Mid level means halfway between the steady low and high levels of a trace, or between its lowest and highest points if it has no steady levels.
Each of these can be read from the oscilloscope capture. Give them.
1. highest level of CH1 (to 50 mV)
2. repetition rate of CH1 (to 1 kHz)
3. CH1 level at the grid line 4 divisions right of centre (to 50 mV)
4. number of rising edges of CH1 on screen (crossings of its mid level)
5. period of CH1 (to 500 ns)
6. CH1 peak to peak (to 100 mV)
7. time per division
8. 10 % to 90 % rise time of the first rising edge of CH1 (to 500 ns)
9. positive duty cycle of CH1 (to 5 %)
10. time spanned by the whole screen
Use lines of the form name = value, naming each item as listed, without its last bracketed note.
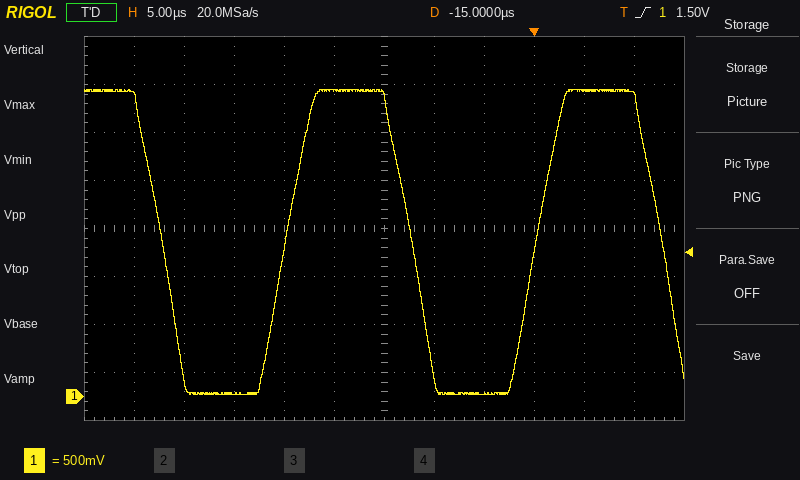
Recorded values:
highest level of CH1 = 3.20 V
repetition rate of CH1 = 40 kHz
CH1 level at the grid line 4 divisions right of centre = 3.20 V
number of rising edges of CH1 on screen = 2
period of CH1 = 25.0 µs
CH1 peak to peak = 3.20 V
time per division = 5 µs
10 % to 90 % rise time of the first rising edge of CH1 = 4.5 µs
positive duty cycle of CH1 = 50 %
time spanned by the whole screen = 60 µs
